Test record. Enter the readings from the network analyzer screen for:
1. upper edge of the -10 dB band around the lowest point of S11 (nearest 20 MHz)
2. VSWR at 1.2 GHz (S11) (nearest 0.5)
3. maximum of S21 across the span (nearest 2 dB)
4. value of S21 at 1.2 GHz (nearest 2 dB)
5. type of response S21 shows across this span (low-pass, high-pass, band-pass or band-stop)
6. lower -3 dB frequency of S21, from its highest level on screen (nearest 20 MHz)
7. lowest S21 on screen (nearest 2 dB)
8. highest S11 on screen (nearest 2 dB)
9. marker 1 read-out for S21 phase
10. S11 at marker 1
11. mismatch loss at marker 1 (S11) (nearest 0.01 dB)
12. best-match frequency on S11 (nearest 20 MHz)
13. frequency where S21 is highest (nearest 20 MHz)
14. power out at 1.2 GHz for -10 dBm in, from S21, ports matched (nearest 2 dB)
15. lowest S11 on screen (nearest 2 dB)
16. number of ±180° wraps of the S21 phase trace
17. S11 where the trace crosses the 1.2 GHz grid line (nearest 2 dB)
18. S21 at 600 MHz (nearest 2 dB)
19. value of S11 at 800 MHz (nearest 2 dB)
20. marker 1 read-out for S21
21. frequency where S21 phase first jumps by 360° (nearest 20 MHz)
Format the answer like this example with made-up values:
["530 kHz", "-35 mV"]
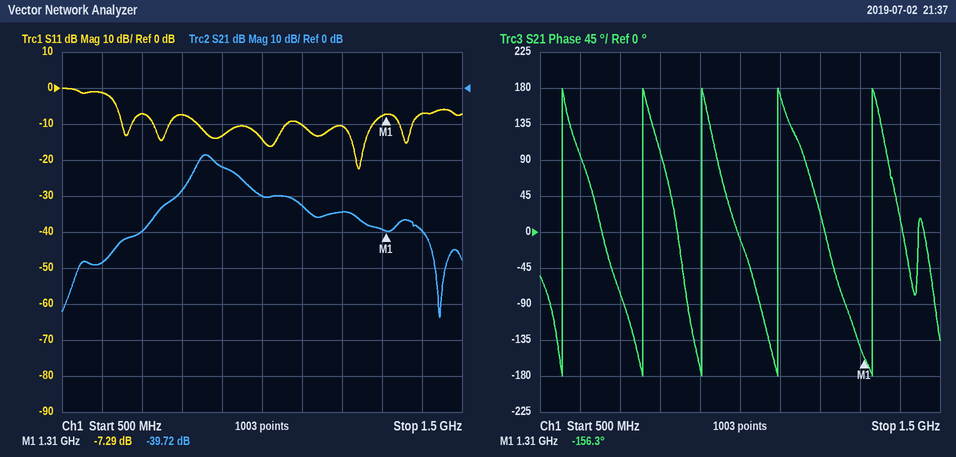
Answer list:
["1.28 GHz", "2.0", "-18 dB", "-34 dB", "band-pass", "840 MHz", "-64 dB", "0 dB", "-156.3°", "-7.29 dB", "0.90 dB", "1.24 GHz", "860 MHz", "-44 dBm", "-22 dB", "5", "-10 dB", "-48 dB", "-8 dB", "-39.72 dB", "560 MHz"]
